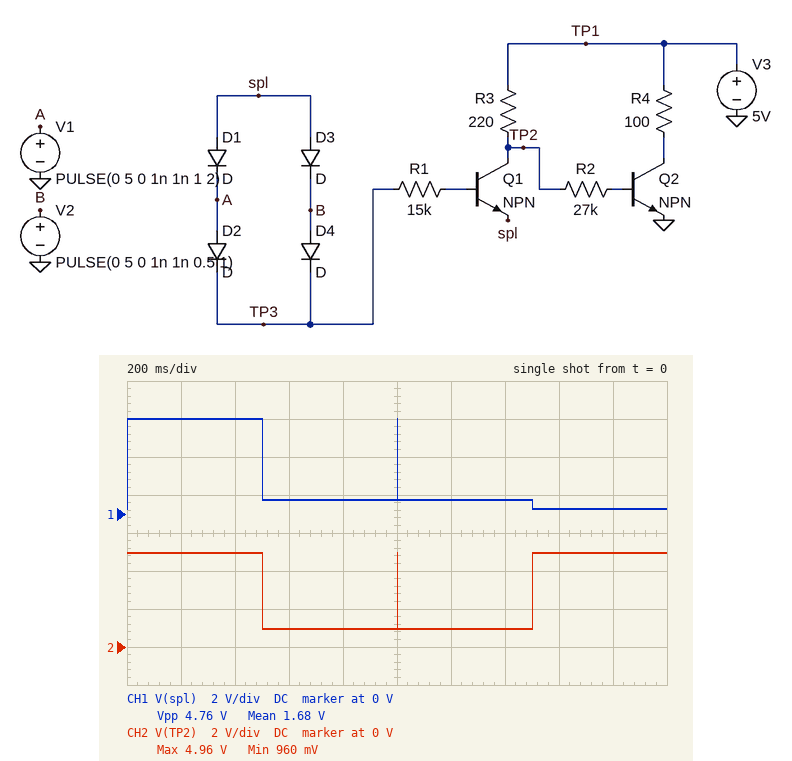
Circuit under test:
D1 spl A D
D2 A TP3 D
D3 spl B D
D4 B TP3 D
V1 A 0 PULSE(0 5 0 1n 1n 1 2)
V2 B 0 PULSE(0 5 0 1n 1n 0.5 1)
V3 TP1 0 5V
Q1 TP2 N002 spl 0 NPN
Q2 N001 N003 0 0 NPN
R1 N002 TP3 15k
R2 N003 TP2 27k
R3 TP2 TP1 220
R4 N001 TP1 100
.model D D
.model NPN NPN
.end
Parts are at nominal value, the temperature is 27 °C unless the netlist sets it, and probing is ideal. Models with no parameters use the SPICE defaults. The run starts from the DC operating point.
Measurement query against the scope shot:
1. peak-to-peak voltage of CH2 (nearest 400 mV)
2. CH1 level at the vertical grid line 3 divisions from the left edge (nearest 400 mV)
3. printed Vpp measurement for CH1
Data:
4.0 V
800 mV
4.76 V
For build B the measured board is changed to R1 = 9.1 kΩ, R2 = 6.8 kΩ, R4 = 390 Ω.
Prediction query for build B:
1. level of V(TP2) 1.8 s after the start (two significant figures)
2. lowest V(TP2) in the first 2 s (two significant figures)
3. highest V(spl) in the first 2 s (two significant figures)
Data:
4.9 V
860 mV
5.0 V
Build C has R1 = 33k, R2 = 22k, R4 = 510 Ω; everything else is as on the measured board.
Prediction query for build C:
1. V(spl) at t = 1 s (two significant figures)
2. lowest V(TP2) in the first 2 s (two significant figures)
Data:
710 mV
3.1 V
